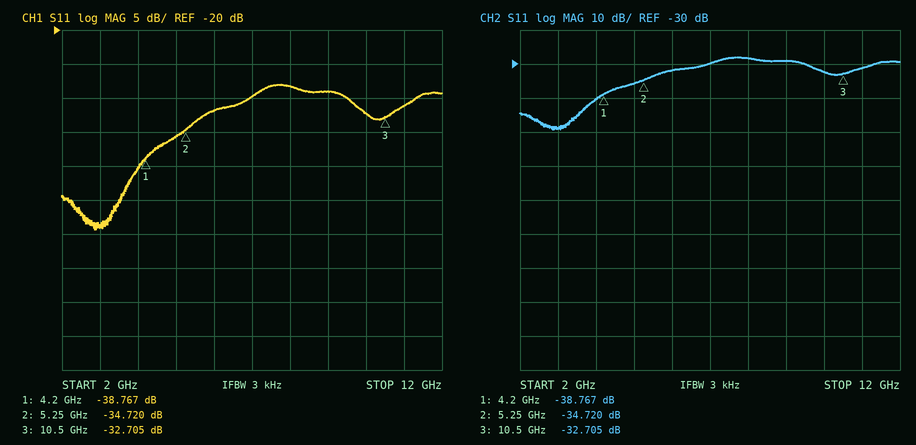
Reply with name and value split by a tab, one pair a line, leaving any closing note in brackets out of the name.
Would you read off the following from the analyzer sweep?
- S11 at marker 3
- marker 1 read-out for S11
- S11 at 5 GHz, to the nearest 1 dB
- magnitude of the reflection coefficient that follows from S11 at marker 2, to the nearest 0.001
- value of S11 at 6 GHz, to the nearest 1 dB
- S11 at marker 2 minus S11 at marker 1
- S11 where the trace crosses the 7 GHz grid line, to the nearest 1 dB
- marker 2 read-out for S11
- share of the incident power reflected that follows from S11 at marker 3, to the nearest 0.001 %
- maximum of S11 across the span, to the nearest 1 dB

S11 at marker 3	-32.705 dB
marker 1 read-out for S11	-38.767 dB
S11 at 5 GHz, to the nearest 1 dB	-36 dB
magnitude of the reflection coefficient that follows from S11 at marker 2, to the nearest 0.001	0.018
value of S11 at 6 GHz, to the nearest 1 dB	-32 dB
S11 at marker 2 minus S11 at marker 1	4.047 dB
S11 where the trace crosses the 7 GHz grid line, to the nearest 1 dB	-30 dB
marker 2 read-out for S11	-34.720 dB
share of the incident power reflected that follows from S11 at marker 3, to the nearest 0.001 %	0.054 %
maximum of S11 across the span, to the nearest 1 dB	-28 dB
